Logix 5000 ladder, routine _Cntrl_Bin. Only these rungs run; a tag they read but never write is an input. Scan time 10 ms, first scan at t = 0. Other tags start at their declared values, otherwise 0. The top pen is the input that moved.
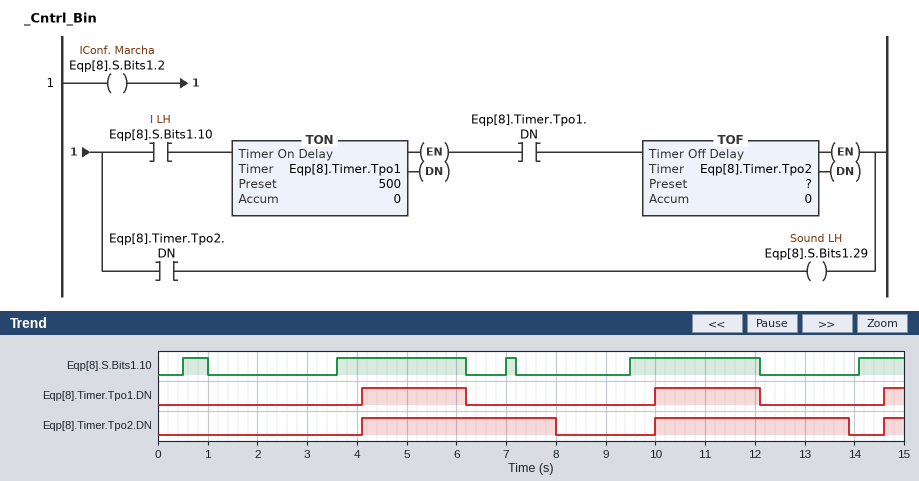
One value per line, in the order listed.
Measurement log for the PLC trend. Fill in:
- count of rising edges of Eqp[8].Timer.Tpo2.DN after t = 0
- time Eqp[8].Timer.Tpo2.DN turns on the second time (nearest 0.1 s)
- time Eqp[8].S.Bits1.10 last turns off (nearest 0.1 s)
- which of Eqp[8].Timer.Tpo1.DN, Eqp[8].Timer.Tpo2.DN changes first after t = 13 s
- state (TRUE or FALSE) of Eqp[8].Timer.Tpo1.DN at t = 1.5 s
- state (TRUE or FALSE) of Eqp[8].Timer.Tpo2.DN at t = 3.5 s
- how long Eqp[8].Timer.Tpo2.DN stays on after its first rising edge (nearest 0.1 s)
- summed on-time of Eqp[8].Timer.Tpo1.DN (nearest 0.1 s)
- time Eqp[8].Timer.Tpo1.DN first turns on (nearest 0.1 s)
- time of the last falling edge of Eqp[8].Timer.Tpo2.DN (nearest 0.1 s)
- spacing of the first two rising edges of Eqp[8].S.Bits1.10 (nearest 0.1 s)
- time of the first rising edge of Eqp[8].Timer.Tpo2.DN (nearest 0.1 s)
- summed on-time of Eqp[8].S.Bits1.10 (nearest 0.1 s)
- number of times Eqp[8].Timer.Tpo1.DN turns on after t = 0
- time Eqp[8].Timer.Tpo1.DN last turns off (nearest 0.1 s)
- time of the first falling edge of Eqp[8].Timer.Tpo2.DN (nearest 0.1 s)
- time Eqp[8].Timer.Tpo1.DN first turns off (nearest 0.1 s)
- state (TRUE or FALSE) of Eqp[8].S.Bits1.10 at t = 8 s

3
10.0 s
12.1 s
Eqp[8].Timer.Tpo2.DN
FALSE
FALSE
3.9 s
4.6 s
4.1 s
13.9 s
3.1 s
4.1 s
6.8 s
3
12.1 s
8.0 s
6.2 s
FALSE
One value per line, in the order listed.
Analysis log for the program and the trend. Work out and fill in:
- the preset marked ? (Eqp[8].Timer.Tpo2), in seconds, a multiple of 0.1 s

1.8 s
